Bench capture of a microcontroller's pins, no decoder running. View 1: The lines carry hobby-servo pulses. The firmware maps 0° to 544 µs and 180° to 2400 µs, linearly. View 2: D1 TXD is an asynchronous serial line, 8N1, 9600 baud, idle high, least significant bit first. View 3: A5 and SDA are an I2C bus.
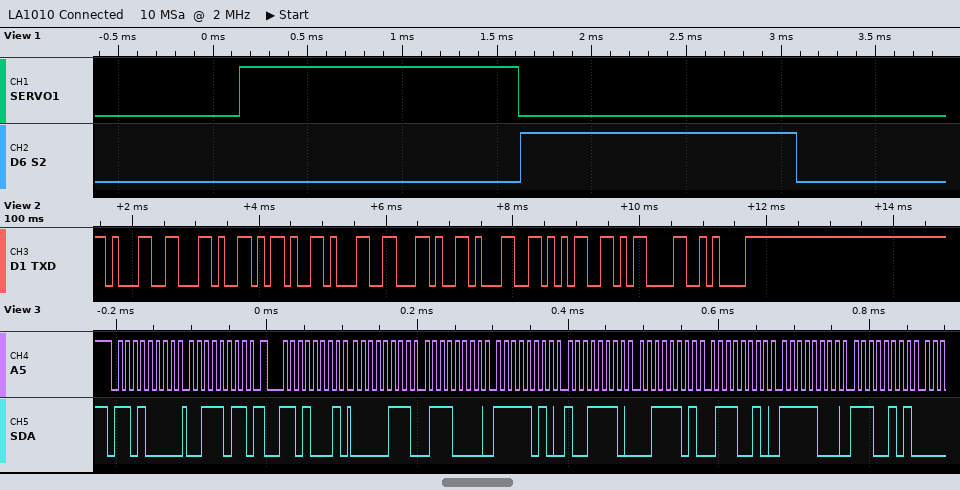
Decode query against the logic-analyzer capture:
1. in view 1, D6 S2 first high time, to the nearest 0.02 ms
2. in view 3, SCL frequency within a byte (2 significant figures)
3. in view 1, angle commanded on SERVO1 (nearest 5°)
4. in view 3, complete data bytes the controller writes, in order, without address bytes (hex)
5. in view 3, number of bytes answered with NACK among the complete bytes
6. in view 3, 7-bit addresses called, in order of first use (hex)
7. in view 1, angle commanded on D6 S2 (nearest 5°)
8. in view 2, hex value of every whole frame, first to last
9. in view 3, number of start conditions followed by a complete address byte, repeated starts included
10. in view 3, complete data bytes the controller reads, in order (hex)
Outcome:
1.46 ms
100 kHz
90°
3B
0
0x68
90°
31 2C 2D 31 2C 31 35 0D 0A
2
07 70 FA 9E 3D 72 F8 E5
